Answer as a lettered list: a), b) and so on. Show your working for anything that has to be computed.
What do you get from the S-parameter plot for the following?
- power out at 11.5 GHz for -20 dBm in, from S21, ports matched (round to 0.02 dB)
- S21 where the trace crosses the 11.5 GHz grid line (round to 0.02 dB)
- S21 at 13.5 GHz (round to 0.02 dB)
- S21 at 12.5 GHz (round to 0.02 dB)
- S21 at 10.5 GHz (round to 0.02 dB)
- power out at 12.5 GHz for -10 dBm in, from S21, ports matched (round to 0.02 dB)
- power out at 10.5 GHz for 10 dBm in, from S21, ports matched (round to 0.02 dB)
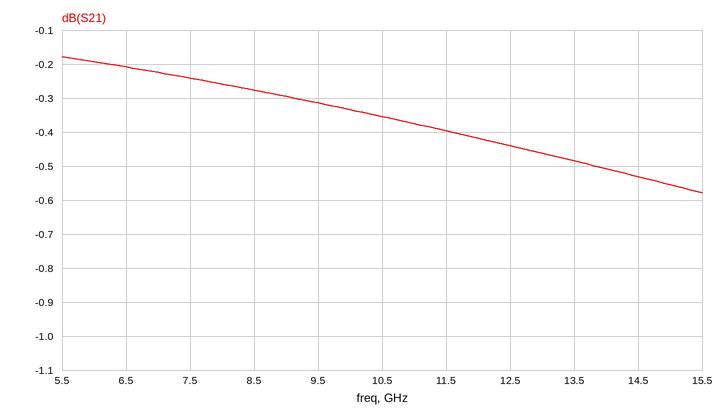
a) -20 dBm + (-0.40 dB) = -20.40 dBm
b) -0.40 dB
c) -0.48 dB
d) -0.44 dB
e) -0.36 dB
f) -10 dBm + (-0.44 dB) = -10.44 dBm
g) 10 dBm + (-0.36 dB) = 9.64 dBm
